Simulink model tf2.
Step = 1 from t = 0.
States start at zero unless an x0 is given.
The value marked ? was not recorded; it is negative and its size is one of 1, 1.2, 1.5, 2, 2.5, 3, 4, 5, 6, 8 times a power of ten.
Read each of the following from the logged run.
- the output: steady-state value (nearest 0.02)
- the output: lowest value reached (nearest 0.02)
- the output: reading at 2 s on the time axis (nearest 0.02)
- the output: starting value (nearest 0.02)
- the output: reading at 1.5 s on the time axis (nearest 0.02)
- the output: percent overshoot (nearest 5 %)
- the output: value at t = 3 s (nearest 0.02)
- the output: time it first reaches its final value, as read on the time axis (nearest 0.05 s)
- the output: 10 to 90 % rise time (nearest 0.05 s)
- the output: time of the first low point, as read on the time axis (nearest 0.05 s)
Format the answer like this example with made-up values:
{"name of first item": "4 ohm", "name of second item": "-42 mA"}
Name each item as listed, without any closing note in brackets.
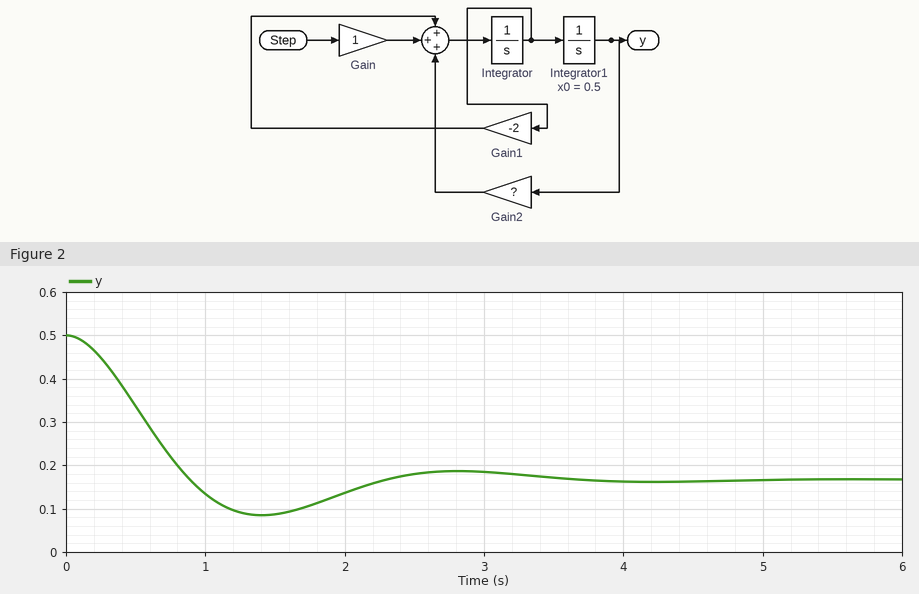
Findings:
{"the output: steady-state value": "0.16", "the output: lowest value reached": "0.08", "the output: reading at 2 s on the time axis": "0.14", "the output: starting value": "0.50", "the output: reading at 1.5 s on the time axis": "0.08", "the output: percent overshoot": "25 %", "the output: value at t = 3 s": "0.18", "the output: time it first reaches its final value, as read on the time axis": "0.90 s", "the output: 10 to 90 % rise time": "0.60 s", "the output: time of the first low point, as read on the time axis": "1.40 s"}
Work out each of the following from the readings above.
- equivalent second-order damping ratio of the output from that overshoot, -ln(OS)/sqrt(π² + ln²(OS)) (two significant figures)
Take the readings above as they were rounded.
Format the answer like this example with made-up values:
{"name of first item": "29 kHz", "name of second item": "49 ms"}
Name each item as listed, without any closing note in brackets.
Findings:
{"equivalent second-order damping ratio of the output from that overshoot, -ln(OS)/sqrt(π² + ln²(OS))": "0.40"}
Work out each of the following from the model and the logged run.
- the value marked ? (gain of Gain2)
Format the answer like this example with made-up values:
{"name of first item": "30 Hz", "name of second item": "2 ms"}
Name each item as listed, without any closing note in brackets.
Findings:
{"the value marked ?": "-6"}
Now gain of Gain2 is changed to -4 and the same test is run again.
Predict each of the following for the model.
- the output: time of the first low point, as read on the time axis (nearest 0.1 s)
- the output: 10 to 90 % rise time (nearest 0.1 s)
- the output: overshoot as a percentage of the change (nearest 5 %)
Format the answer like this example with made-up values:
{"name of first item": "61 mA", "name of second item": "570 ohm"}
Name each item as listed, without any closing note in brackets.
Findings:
{"the output: time of the first low point, as read on the time axis": "1.8 s", "the output: 10 to 90 % rise time": "0.8 s", "the output: overshoot as a percentage of the change": "15 %"}
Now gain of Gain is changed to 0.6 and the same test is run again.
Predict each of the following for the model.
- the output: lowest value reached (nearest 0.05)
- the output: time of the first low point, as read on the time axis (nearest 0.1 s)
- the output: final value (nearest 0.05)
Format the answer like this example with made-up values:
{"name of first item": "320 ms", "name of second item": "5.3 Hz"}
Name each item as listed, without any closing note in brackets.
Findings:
{"the output: lowest value reached": "0.00", "the output: time of the first low point, as read on the time axis": "1.4 s", "the output: final value": "0.10"}
